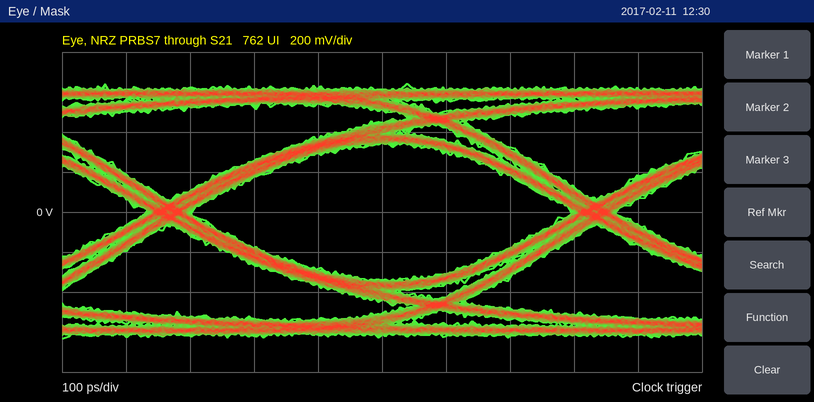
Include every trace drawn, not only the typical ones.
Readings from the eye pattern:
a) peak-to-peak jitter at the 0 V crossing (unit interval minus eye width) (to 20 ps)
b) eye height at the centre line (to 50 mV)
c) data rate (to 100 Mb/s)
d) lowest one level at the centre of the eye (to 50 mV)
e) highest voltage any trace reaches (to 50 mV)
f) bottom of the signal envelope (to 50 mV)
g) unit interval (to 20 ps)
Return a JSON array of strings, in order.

["80 ps", "700 mV", "1.5 Gb/s", "350 mV", "650 mV", "-650 mV", "660 ps"]
